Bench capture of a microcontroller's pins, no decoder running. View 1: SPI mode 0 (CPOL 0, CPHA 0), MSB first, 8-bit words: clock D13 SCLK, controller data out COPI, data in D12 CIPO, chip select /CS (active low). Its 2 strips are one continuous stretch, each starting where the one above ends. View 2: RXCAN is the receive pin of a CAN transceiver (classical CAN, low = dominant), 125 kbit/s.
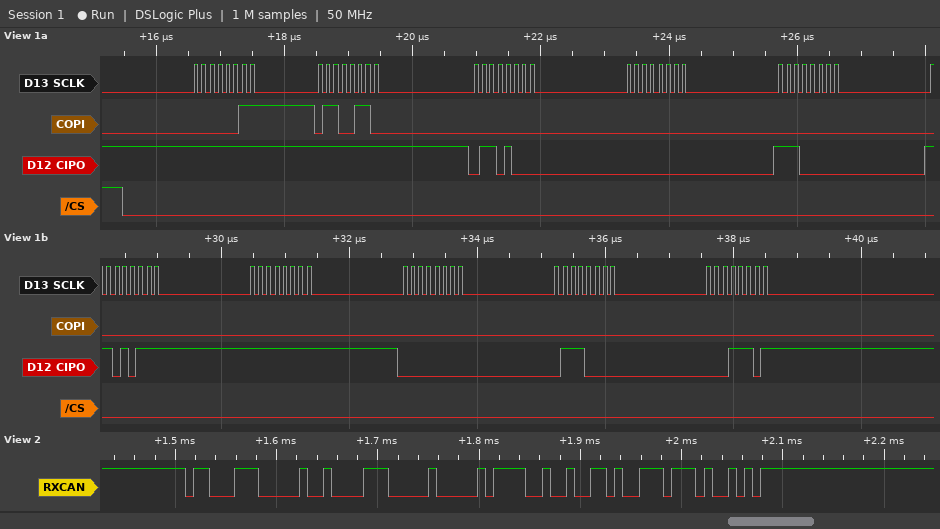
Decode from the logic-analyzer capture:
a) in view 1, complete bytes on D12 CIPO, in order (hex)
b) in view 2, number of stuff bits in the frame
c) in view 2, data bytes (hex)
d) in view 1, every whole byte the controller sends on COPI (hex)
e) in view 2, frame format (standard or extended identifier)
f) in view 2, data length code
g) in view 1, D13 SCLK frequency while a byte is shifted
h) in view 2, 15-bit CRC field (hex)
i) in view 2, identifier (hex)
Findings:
FF FF 68 00 E0 D7 FF 00 70 1D
3
38 00 F2 4D
03 66 00 00 00 00 00 00 00 00
standard
4
8 MHz
0x1DD2
0x638
